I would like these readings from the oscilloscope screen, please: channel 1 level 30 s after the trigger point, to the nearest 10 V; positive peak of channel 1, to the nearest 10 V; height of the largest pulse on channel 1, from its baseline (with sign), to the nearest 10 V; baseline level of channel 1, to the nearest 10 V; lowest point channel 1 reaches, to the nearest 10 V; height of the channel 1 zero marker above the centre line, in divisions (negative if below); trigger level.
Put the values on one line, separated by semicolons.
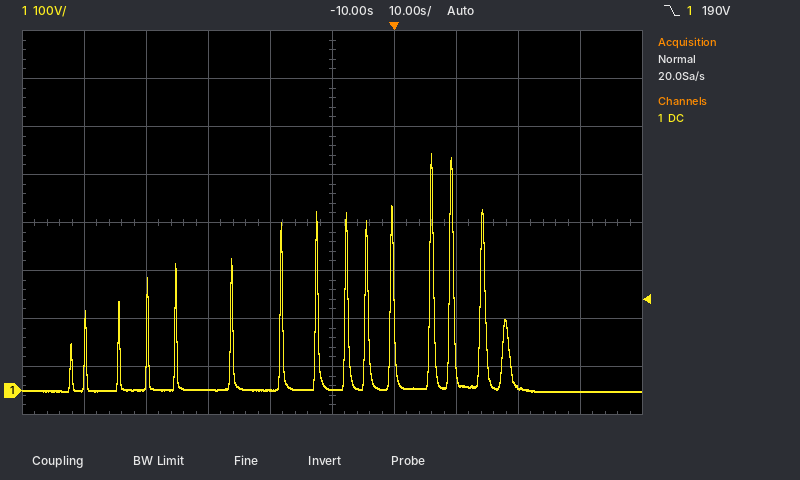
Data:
0 V; 490 V; +490 V; 0 V; 0 V; -3.5 div; 190 V
